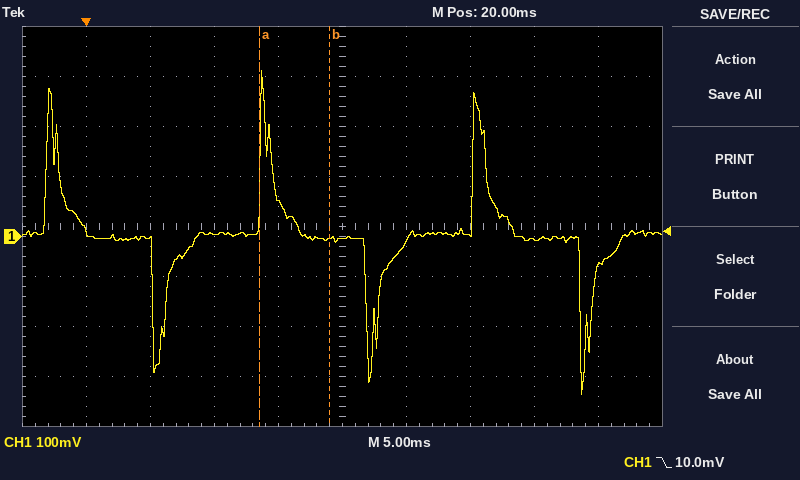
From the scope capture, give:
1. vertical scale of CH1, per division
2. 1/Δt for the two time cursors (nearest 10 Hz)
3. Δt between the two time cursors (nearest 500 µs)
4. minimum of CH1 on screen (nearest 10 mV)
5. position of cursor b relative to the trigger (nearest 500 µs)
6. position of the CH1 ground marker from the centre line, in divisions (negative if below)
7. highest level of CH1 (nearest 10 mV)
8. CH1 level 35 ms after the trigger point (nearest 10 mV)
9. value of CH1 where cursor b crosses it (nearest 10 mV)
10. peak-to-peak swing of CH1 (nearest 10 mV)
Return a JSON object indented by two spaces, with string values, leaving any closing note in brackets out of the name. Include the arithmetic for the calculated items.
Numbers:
{
  "vertical scale of CH1, per division": "100 mV",
  "1/Δt for the two time cursors": "1 / 5.5 ms ≈ 180 Hz",
  "Δt between the two time cursors": "5.5 ms",
  "minimum of CH1 on screen": "-320 mV",
  "position of cursor b relative to the trigger": "+19.0 ms",
  "position of the CH1 ground marker from the centre line, in divisions": "-0.2 div",
  "highest level of CH1": "330 mV",
  "CH1 level 35 ms after the trigger point": "-10 mV",
  "value of CH1 where cursor b crosses it": "0 mV",
  "peak-to-peak swing of CH1": "330 mV − (-320 mV) = 650 mV"
}
